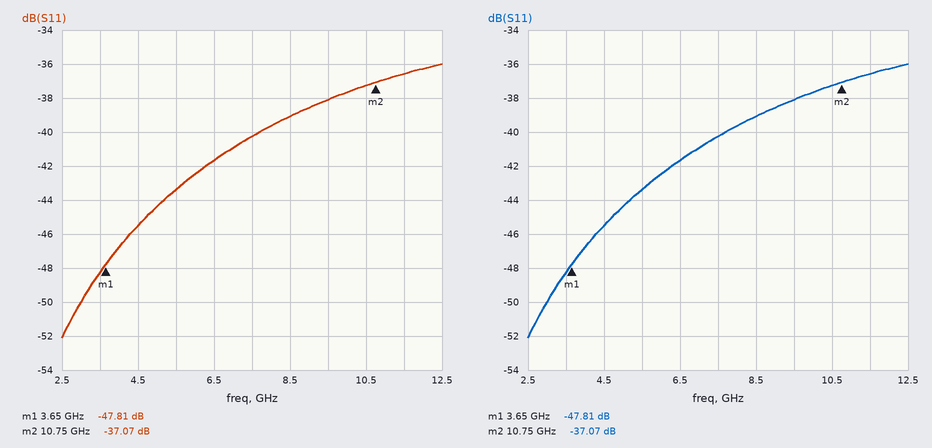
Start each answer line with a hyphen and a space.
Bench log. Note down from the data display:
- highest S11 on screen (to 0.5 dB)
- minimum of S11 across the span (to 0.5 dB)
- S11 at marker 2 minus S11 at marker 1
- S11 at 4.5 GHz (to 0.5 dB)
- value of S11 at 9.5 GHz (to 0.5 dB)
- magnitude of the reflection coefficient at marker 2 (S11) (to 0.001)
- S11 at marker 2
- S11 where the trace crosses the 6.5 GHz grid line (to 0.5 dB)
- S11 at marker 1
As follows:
- -36.0 dB
- -52.0 dB
- 10.74 dB
- -45.5 dB
- -38.0 dB
- 0.014
- -37.07 dB
- -41.5 dB
- -47.81 dB
